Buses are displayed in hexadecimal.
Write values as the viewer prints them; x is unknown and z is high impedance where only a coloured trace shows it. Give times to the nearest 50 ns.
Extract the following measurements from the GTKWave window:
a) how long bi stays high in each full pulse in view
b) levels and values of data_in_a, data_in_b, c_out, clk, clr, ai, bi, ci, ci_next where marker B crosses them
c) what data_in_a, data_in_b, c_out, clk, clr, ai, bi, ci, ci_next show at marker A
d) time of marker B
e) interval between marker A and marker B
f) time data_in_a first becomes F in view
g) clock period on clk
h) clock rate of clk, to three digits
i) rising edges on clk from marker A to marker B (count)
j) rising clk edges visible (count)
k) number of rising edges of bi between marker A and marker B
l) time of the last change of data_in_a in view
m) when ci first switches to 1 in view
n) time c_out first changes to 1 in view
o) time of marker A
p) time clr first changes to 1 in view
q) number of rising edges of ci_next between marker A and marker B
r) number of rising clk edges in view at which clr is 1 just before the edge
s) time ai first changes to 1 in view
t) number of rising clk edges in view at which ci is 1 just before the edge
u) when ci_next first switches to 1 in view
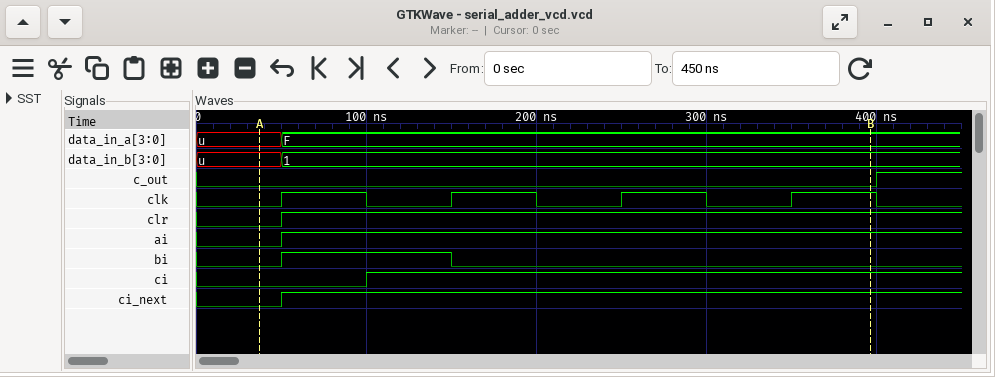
100 ns
data_in_a=F, data_in_b=1, c_out=0, clk=1, clr=1, ai=1, bi=0, ci=1, ci_next=1
data_in_a=u, data_in_b=u, c_out=0, clk=0, clr=0, ai=0, bi=0, ci=0, ci_next=0
400 ns
350 ns
50 ns
100 ns
10.0 MHz
4
4
1
50 ns
100 ns
400 ns
50 ns
50 ns
1
3
50 ns
3
50 ns
